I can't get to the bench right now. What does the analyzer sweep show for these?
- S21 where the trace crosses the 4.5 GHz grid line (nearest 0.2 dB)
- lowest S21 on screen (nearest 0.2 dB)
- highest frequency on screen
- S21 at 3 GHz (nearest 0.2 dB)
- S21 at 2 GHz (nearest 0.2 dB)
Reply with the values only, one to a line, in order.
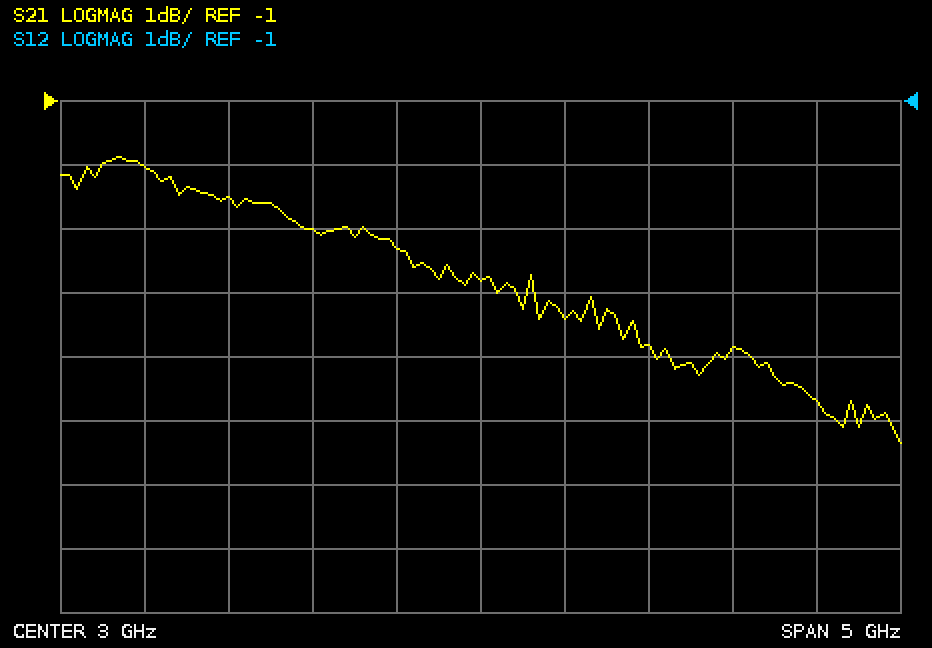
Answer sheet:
-4.8 dB
-6.4 dB
5.5 GHz
-3.8 dB
-3.0 dB
